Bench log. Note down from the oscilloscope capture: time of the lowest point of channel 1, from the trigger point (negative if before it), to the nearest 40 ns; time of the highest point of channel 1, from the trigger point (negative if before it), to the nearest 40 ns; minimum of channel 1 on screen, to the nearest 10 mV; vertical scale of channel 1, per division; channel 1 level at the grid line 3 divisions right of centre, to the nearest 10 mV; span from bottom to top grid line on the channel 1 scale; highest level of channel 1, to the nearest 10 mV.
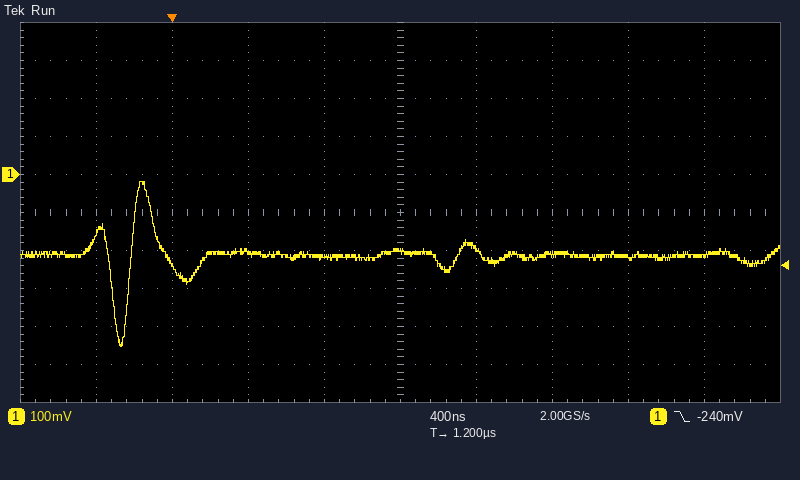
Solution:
-280 ns
-160 ns
-450 mV
100 mV
-220 mV
1 V
-20 mV
